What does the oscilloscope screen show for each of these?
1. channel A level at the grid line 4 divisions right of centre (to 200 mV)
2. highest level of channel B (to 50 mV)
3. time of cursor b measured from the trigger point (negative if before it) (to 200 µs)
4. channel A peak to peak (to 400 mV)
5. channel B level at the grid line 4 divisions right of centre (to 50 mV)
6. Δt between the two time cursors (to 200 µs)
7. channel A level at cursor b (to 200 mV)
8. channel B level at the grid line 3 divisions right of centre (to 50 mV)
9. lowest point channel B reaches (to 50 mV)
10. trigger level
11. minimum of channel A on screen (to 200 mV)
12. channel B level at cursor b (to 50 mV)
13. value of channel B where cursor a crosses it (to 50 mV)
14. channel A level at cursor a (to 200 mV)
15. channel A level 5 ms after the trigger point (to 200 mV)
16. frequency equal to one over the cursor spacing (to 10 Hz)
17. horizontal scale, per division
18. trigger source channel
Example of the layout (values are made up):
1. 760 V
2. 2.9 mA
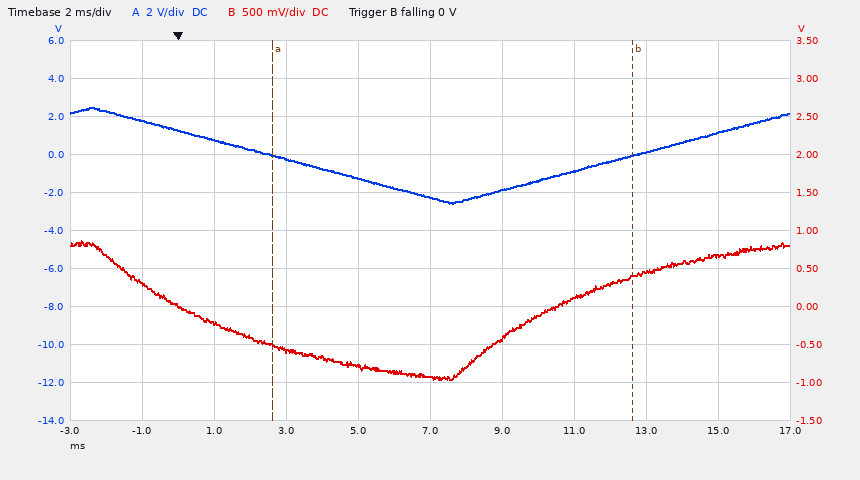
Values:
1. 1.2 V
2. 850 mV
3. +12.6 ms
4. 5.2 V
5. 650 mV
6. 10.0 ms
7. 0.0 V
8. 450 mV
9. -950 mV
10. 0 V
11. -2.6 V
12. 400 mV
13. -500 mV
14. 0.0 V
15. -1.2 V
16. 100 Hz
17. 2 ms
18. channel B
